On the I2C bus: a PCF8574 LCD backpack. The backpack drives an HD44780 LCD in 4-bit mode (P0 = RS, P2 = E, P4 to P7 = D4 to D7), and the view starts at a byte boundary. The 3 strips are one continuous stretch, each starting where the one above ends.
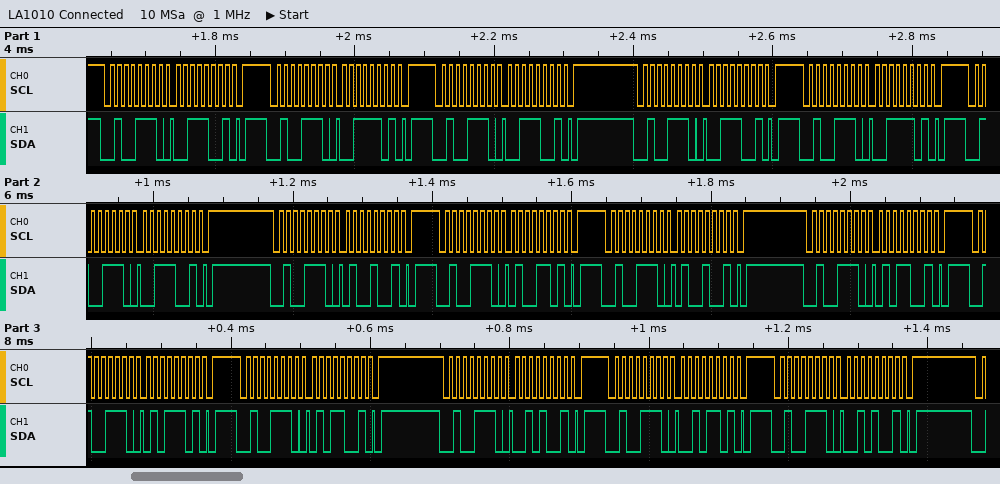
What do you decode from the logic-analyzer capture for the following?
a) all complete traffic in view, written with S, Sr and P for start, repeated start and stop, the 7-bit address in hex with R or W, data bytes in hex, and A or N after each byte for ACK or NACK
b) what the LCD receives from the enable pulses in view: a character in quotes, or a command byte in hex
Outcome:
S 27W A 39 A P S 27W A 3D A P S 27W A 39 A P S 27W A 39 A P S 27W A 3D A P S 27W A 39 A P S 27W A 49 A P S 27W A 4D A P S 27W A 49 A P S 27W A 59 A P S 27W A 5D A P S 27W A 59 A P S 27W A 29 A P S 27W A 2D A P S 27W A 29 A P
'3' 'E'
